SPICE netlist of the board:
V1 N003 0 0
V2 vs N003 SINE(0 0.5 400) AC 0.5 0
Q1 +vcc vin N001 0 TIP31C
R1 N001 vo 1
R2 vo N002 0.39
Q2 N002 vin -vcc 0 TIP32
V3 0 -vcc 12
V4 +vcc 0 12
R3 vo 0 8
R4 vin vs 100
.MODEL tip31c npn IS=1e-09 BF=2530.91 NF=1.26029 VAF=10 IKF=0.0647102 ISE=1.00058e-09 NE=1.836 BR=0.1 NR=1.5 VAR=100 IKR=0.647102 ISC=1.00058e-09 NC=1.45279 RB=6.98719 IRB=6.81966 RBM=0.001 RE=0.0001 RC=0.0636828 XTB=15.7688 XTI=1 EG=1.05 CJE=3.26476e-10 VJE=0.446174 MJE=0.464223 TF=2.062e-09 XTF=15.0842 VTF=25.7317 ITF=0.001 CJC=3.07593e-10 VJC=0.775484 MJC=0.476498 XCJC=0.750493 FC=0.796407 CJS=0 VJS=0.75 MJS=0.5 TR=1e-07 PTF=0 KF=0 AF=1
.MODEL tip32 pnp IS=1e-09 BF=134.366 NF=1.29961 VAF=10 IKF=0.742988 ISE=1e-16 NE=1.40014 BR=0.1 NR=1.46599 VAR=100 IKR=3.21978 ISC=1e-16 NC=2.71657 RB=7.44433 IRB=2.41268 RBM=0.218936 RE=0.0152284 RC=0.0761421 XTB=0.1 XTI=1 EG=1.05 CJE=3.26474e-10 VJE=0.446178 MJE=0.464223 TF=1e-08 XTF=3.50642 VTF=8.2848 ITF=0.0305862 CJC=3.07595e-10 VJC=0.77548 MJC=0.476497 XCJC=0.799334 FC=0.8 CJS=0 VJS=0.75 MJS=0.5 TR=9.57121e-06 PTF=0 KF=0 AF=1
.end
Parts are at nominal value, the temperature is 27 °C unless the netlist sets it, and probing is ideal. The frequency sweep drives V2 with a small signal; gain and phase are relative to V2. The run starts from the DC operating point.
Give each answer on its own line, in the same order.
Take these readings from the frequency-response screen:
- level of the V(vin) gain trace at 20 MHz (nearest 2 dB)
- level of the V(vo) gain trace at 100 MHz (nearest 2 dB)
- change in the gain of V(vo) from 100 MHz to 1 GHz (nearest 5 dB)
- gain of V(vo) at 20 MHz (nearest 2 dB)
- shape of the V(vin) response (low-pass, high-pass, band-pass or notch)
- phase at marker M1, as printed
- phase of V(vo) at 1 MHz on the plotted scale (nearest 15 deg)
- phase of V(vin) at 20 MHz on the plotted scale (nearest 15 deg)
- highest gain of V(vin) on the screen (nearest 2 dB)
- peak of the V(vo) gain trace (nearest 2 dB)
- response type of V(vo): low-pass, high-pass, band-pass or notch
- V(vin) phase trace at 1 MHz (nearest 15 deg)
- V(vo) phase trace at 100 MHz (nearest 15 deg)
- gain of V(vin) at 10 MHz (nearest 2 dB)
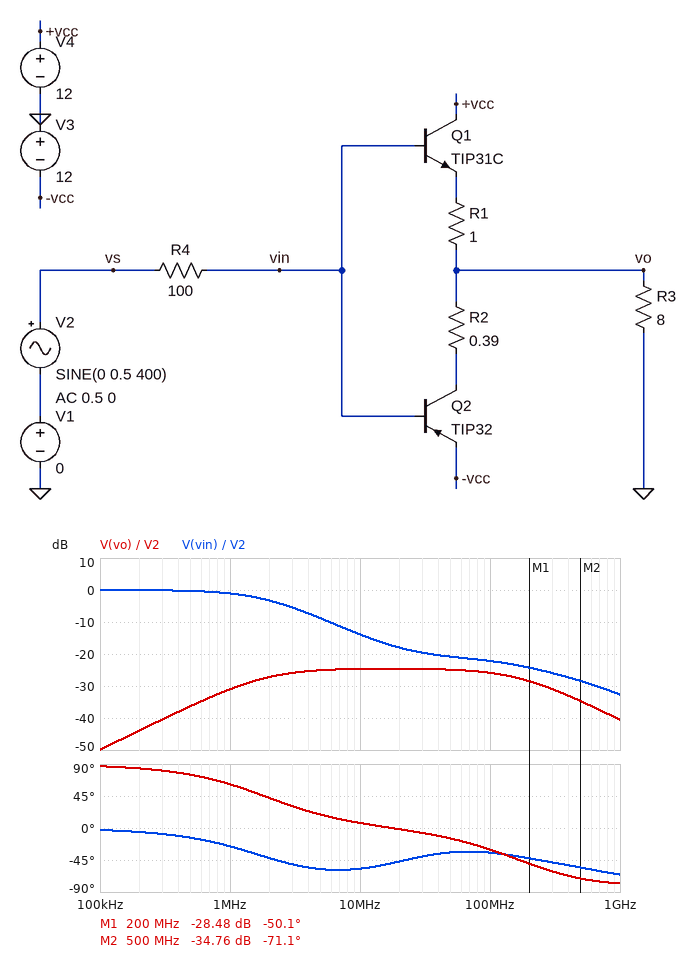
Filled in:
-18 dB
-26 dB
-15 dB
-24 dB
low-pass
-50.1 deg
60 deg
-45 deg
0 dB
-24 dB
band-pass
-30 deg
-30 deg
-14 dB
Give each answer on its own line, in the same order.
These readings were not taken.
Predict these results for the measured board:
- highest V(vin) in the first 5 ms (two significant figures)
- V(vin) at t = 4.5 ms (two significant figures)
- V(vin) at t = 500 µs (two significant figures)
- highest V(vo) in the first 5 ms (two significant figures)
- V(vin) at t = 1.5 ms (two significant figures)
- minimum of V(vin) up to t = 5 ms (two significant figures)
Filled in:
500 mV
-420 mV
470 mV
28 mV
-290 mV
-430 mV
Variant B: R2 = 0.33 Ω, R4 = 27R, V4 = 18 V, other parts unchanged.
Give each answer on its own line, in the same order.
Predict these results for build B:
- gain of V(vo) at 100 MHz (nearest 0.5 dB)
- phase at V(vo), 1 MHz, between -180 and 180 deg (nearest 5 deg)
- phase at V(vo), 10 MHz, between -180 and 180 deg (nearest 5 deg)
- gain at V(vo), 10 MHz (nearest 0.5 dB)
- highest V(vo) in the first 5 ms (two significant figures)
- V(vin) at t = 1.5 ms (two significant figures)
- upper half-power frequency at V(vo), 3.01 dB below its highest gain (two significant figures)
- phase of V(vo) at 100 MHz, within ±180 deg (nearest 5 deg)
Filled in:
-15.5 dB
80 deg
25 deg
-16.0 dB
32 mV
-290 mV
220 MHz
-20 deg
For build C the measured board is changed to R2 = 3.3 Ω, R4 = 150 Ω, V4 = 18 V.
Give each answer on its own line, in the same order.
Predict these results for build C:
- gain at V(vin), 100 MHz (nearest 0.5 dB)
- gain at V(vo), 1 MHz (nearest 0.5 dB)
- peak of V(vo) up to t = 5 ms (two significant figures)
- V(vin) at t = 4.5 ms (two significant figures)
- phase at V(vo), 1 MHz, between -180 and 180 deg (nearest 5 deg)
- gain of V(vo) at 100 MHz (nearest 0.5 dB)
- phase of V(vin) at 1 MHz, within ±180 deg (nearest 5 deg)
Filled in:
-25.0 dB
-32.0 dB
31 mV
-410 mV
50 deg
-29.0 dB
-35 deg
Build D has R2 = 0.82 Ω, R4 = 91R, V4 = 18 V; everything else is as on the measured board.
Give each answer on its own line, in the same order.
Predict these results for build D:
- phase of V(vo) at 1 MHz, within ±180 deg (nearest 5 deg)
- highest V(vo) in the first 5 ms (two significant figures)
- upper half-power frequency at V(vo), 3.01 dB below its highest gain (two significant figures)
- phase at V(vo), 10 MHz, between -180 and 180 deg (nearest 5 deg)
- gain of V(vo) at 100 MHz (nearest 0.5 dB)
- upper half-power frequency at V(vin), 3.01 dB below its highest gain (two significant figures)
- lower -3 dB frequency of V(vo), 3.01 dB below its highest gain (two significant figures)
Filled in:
65 deg
32 mV
180 MHz
10 deg
-25.0 dB
2.1 MHz
2.0 MHz
